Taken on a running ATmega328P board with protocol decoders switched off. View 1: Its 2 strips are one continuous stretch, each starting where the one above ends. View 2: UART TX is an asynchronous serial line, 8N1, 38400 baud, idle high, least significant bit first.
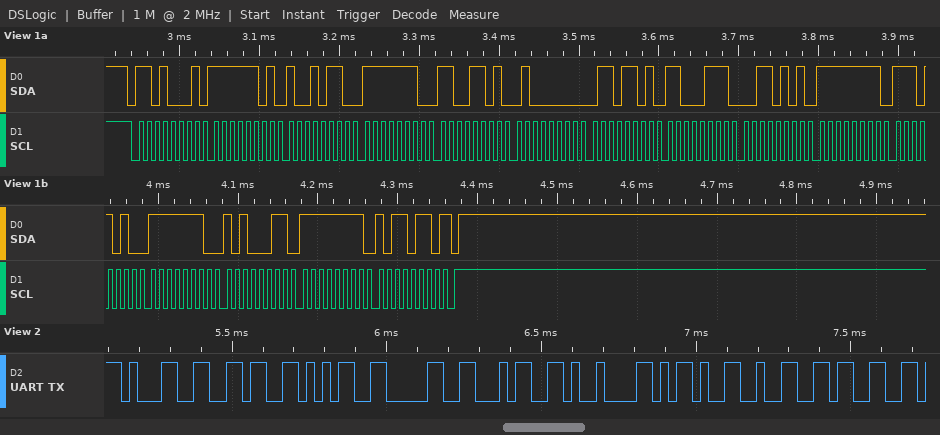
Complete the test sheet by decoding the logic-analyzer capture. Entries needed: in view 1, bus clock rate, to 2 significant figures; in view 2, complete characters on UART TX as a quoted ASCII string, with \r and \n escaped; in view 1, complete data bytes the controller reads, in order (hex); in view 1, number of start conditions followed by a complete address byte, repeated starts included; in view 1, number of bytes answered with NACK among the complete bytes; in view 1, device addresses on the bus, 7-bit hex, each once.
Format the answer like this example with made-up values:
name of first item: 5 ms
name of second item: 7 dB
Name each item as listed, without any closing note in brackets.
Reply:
in view 1, bus clock rate, to 2 significant figures: 100 kHz
in view 2, complete characters on UART TX as a quoted ASCII string, with \r and \n escaped: "16504\t-23"
in view 1, complete data bytes the controller reads, in order: FD 96 FE CD 40 6D C7 35 FF EA FE A3 FF B6
in view 1, number of start conditions followed by a complete address byte, repeated starts included: 1
in view 1, number of bytes answered with NACK among the complete bytes: 1
in view 1, device addresses on the bus, 7-bit hex, each once: 0x68
